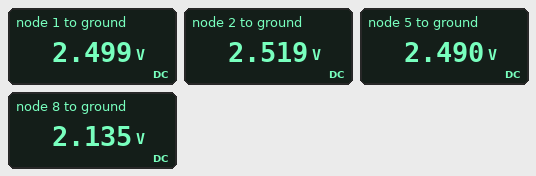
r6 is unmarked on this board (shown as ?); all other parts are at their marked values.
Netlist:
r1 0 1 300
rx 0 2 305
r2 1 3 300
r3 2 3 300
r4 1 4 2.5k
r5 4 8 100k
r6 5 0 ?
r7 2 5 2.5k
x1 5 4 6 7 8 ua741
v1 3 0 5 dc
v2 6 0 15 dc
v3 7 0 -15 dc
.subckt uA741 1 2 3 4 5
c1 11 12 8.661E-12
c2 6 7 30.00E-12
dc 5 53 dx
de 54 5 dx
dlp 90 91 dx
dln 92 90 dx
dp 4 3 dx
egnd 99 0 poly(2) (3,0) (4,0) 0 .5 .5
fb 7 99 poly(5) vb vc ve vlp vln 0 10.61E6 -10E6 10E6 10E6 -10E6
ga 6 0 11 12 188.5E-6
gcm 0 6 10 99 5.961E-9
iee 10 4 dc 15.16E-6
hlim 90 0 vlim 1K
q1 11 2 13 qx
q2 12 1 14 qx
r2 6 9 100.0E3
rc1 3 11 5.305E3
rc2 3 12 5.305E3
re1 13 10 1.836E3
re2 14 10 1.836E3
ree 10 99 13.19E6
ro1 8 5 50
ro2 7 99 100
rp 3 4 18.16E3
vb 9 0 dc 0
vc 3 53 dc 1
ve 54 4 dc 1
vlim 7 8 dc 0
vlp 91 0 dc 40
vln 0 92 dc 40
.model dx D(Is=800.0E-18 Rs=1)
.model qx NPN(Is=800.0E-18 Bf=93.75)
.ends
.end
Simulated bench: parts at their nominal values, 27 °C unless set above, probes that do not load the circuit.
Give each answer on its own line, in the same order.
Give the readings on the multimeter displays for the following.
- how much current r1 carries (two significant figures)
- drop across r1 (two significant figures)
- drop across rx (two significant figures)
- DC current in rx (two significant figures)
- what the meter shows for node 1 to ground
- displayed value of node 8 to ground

8.3 mA
2.5 V
2.5 V
8.3 mA
2.499 V
2.135 V
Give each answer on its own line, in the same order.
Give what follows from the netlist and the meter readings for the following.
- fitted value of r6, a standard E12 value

220 kΩ
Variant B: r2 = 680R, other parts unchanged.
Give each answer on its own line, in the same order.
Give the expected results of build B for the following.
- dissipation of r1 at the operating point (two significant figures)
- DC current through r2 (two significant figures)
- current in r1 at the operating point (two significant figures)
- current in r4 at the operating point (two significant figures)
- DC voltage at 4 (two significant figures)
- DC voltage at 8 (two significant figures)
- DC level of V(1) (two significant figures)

8.1 mW
5.1 mA
5.2 mA
130 µA
1.9 V
15 V
1.6 V
